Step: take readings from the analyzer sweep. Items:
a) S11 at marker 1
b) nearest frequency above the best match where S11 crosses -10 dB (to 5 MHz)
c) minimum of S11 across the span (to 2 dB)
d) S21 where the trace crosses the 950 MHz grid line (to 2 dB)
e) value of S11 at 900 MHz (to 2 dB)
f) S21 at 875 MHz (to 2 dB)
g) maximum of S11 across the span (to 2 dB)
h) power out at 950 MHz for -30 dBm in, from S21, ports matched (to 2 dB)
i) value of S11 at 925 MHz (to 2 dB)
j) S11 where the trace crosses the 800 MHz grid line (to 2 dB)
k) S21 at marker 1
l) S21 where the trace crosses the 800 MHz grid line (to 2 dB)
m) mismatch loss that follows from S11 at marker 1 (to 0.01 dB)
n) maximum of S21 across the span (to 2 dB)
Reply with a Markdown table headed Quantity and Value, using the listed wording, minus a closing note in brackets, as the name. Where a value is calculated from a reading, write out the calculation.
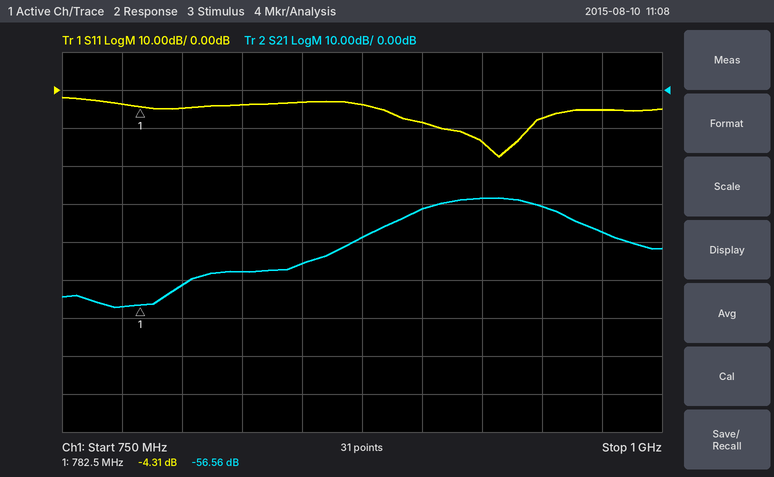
| Quantity | Value |
|---|---|
| S11 at marker 1 | -4.31 dB |
| nearest frequency above the best match where S11 crosses -10 dB | 945 MHz |
| minimum of S11 across the span | -18 dB |
| S21 where the trace crosses the 950 MHz grid line | -30 dB |
| value of S11 at 900 MHz | -8 dB |
| S21 at 875 MHz | -38 dB |
| maximum of S11 across the span | -2 dB |
| power out at 950 MHz for -30 dBm in, from S21, ports matched | -30 dBm + (-30 dB) = -60 dBm |
| value of S11 at 925 MHz | -14 dB |
| S11 where the trace crosses the 800 MHz grid line | -4 dB |
| S21 at marker 1 | -56.56 dB |
| S21 where the trace crosses the 800 MHz grid line | -52 dB |
| mismatch loss that follows from S11 at marker 1 | −10 log10(1 − 10^(-4.31/10)) ≈ 2.01 dB |
| maximum of S21 across the span | -28 dB |
